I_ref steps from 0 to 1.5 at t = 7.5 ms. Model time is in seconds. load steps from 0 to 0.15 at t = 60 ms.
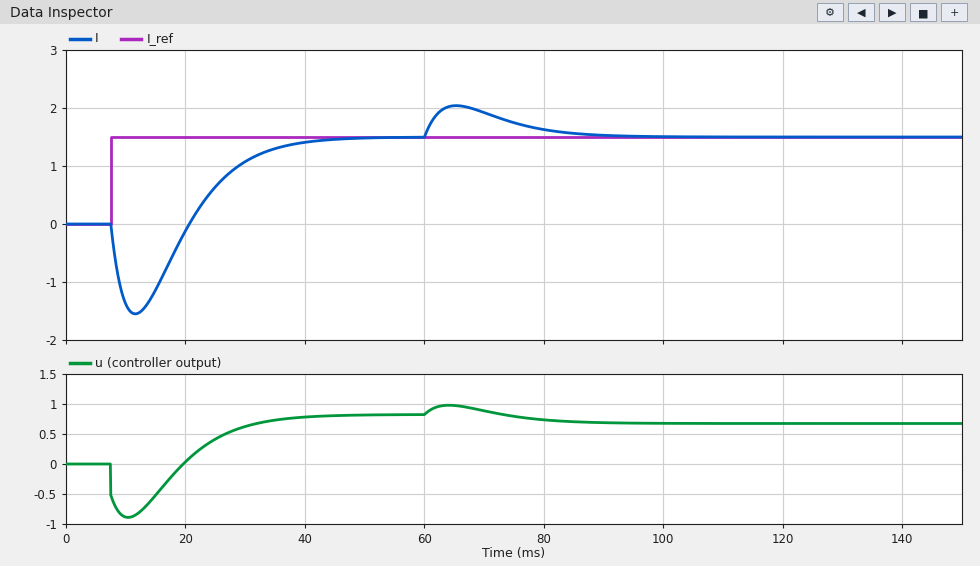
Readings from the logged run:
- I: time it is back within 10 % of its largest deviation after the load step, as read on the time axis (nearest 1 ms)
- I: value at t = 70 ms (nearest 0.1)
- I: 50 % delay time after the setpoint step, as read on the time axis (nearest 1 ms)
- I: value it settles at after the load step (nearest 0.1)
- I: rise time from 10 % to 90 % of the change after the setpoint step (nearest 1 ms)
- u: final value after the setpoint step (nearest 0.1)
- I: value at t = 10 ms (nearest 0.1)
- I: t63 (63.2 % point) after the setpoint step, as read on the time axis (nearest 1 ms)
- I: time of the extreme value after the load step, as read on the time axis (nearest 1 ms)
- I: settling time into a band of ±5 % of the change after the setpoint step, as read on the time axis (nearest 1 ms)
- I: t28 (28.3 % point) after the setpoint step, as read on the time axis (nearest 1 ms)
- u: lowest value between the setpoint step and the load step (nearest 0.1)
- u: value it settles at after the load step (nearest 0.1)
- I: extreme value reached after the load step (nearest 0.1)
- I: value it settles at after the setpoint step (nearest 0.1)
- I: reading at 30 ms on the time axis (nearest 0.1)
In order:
86 ms
1.9
26 ms
1.5
15 ms
0.8
-1.4
28 ms
65 ms
41 ms
23 ms
-0.9
0.7
2.0
1.5
1.1
